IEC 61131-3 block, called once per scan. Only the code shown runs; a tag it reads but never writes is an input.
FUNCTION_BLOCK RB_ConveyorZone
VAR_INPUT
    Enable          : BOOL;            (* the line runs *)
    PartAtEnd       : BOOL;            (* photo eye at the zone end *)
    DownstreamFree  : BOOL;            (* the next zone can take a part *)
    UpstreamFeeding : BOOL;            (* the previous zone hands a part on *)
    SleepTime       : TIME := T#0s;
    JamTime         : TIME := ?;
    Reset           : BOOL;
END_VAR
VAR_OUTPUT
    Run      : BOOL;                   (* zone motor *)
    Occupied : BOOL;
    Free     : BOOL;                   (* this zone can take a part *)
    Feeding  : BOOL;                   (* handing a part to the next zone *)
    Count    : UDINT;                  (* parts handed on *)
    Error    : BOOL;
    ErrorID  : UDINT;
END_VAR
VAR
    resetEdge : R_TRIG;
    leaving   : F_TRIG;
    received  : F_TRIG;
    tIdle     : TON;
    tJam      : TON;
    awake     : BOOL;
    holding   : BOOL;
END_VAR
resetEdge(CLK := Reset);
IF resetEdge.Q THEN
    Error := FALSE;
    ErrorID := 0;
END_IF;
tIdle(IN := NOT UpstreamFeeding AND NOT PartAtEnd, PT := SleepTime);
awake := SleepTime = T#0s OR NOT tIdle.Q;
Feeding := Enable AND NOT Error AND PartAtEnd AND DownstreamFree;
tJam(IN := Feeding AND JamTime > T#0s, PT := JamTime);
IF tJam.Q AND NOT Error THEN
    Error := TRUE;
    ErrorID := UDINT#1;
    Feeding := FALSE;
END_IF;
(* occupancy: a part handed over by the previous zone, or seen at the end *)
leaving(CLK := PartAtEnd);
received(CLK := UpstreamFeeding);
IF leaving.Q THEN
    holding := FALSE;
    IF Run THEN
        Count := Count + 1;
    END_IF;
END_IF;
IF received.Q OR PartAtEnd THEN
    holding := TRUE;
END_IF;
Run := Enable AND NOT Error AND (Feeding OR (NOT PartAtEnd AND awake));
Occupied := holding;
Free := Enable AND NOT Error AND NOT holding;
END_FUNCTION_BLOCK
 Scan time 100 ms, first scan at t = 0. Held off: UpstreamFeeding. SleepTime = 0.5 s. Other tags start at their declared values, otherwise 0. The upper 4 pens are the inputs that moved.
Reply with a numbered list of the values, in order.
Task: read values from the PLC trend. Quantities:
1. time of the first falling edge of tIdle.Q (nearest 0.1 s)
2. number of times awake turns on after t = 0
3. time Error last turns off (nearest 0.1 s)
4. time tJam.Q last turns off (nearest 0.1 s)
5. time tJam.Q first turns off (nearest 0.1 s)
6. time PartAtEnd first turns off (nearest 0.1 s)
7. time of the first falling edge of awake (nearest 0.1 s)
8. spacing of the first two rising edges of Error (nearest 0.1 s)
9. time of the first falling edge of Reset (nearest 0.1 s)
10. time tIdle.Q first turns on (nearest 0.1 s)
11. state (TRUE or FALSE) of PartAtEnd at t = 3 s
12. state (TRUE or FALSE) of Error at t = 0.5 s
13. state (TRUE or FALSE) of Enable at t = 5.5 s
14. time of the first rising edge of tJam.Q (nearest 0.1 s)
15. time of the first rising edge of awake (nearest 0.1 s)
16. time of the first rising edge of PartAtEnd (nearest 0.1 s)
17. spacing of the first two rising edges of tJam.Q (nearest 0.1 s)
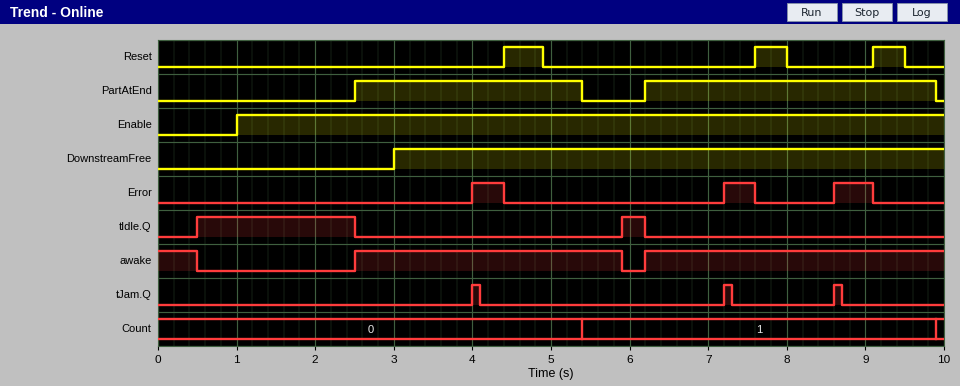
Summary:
1. 2.5 s
2. 2
3. 9.1 s
4. 8.7 s
5. 4.1 s
6. 5.4 s
7. 0.5 s
8. 3.2 s
9. 4.9 s
10. 0.5 s
11. TRUE
12. FALSE
13. TRUE
14. 4.0 s
15. 2.5 s
16. 2.5 s
17. 3.2 s
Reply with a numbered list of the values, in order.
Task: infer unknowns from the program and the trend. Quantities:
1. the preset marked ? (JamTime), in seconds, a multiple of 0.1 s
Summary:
1. 1.0 s
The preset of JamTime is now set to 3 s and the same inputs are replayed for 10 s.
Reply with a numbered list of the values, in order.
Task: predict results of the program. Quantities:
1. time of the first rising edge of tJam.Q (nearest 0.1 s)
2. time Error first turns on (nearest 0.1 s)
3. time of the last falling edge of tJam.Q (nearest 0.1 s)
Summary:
1. 9.2 s
2. 9.2 s
3. 9.3 s
